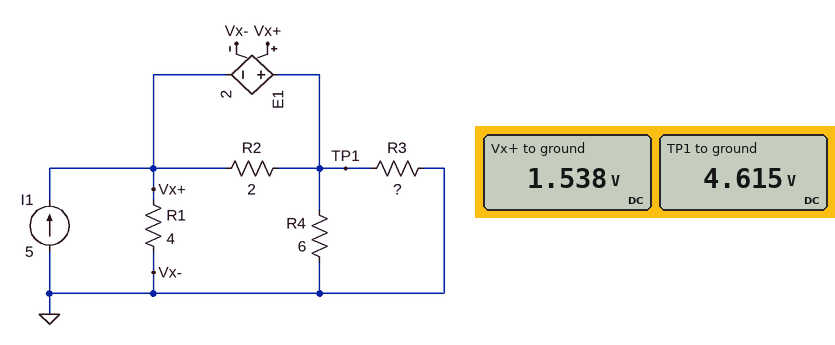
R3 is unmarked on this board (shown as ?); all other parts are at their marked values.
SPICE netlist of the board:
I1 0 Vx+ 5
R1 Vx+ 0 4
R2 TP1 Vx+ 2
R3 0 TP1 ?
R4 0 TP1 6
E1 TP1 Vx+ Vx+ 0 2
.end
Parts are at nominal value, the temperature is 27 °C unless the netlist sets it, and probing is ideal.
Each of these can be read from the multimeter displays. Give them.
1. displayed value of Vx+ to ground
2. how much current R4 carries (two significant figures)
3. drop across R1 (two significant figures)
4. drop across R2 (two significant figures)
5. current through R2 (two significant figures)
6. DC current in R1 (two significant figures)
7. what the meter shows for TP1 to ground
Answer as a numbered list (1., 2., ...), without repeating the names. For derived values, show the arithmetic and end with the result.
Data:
1. 1.538 V
2. (4.615 V) / 6 Ω = 770 mA
3. 1.538 V = 1.5 V
4. 4.615 V - 1.538 V = 3.1 V
5. (4.615 V - 1.538 V) / 2 Ω = 1.5 A
6. (1.538 V) / 4 Ω = 380 mA
7. 4.615 V
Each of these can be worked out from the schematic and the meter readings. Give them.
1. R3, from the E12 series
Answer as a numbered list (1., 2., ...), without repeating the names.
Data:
1. 1.2 Ω
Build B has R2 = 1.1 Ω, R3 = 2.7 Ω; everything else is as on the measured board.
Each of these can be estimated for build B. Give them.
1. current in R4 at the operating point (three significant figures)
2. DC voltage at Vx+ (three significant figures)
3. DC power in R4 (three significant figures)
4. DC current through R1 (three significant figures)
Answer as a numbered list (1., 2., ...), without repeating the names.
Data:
1. 1.34 A
2. 2.69 V
3. 10.8 W
4. 672 mA
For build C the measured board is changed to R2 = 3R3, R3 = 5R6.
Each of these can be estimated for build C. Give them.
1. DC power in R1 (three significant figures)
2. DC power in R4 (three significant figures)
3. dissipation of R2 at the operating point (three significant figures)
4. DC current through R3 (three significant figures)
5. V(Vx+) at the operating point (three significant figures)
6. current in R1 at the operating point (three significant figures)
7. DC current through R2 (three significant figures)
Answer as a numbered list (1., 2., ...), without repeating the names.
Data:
1. 3.78 W
2. 22.7 W
3. 18.3 W
4. 2.08 A
5. 3.89 V
6. 972 mA
7. 2.36 A
